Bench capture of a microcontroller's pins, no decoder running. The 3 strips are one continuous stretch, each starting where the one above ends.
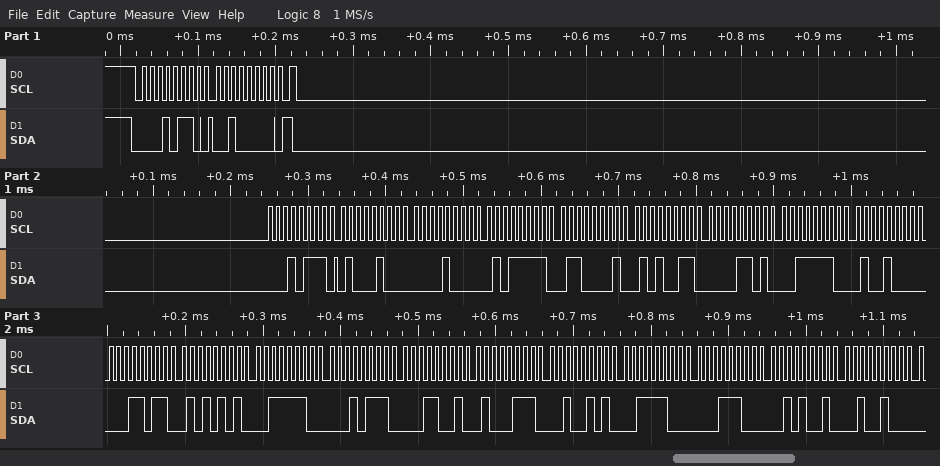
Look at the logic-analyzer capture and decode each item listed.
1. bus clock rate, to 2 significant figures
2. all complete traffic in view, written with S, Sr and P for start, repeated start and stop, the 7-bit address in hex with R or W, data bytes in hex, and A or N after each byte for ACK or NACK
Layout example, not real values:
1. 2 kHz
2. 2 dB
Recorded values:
1. 100 kHz
2. S 0BW A 20 A Sr 0BR A 44 A 08 A 5F A 61 A 53 A 0D A 3E A 48 A 1B A 55 A 3E A 17 A 19 A 47 A 25 A 3C A 1C A 29 A 24 A
